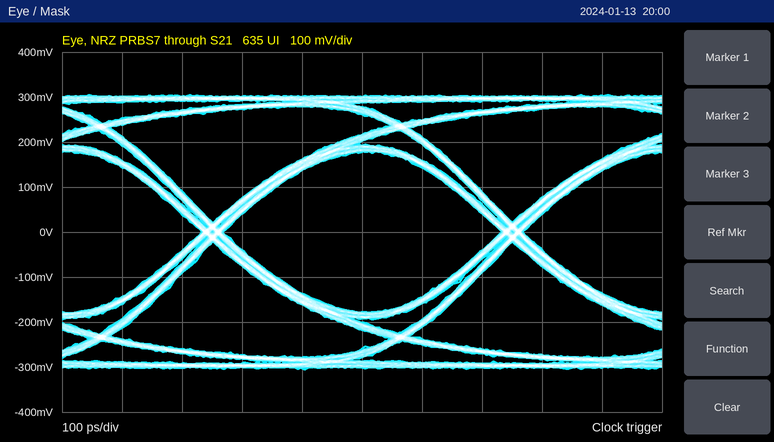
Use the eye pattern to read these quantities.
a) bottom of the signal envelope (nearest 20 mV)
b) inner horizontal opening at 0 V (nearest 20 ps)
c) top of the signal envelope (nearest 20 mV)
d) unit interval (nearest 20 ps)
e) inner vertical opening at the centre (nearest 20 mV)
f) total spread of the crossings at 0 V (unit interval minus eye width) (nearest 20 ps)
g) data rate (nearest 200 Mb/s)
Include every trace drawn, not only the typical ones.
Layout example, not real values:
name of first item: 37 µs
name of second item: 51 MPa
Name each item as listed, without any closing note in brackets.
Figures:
bottom of the signal envelope: -300 mV
inner horizontal opening at 0 V: 460 ps
top of the signal envelope: 300 mV
unit interval: 500 ps
inner vertical opening at the centre: 360 mV
total spread of the crossings at 0 V (unit interval minus eye width): 40 ps
data rate: 2.0 Gb/s
